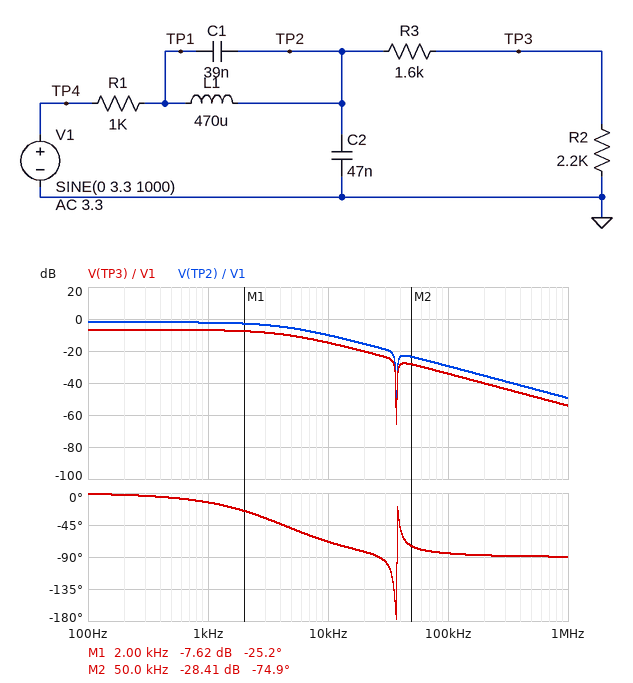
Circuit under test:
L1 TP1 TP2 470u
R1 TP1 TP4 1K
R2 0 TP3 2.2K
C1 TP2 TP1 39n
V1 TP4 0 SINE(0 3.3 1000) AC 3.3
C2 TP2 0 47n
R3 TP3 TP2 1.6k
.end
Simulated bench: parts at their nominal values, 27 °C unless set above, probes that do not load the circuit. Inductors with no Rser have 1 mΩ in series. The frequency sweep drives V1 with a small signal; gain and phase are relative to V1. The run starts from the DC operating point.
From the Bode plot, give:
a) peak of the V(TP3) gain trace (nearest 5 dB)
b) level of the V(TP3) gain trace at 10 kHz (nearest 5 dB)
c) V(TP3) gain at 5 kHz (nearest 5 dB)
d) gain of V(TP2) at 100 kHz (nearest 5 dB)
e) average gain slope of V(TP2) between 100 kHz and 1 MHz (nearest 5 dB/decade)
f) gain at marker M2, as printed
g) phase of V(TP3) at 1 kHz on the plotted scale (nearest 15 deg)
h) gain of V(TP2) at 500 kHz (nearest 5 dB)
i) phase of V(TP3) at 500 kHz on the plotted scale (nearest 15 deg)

-5 dB
-15 dB
-10 dB
-30 dB
-20 dB/decade
-28.41 dB
-15 deg
-45 dB
-90 deg
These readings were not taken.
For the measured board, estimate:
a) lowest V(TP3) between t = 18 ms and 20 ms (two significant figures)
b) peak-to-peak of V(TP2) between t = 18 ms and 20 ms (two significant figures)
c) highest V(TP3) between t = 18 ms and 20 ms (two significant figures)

-1.5 V
5.1 V
1.5 V
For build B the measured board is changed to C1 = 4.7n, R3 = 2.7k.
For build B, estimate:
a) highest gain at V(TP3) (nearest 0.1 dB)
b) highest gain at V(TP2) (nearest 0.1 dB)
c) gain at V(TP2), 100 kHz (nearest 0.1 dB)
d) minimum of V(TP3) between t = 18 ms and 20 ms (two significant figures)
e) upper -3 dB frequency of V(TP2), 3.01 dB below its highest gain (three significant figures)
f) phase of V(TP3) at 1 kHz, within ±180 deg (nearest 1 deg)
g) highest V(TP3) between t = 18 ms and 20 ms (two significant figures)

-8.6 dB
-1.6 dB
-37.3 dB
-1.2 V
4.12 kHz
-14 deg
1.2 V
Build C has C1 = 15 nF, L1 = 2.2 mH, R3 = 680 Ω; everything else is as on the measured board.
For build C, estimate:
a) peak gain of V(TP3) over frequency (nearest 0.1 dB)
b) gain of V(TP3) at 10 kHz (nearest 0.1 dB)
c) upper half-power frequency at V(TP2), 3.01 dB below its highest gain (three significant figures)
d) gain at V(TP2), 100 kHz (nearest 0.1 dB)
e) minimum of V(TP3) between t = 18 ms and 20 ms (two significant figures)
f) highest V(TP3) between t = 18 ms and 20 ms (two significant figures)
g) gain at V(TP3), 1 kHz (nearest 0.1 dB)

-4.9 dB
-12.3 dB
4.79 kHz
-29.5 dB
-1.8 V
1.8 V
-5.1 dB
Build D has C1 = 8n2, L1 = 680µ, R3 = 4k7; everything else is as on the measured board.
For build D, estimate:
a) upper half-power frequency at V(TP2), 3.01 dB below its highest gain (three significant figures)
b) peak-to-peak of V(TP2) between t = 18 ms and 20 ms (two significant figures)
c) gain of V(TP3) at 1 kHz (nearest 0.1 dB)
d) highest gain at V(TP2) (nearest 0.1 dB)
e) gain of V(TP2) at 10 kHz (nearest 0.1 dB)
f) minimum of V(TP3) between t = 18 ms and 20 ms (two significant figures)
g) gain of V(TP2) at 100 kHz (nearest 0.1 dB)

3.93 kHz
5.6 V
-11.4 dB
-1.2 dB
-9.9 dB
-890 mV
-30.0 dB
